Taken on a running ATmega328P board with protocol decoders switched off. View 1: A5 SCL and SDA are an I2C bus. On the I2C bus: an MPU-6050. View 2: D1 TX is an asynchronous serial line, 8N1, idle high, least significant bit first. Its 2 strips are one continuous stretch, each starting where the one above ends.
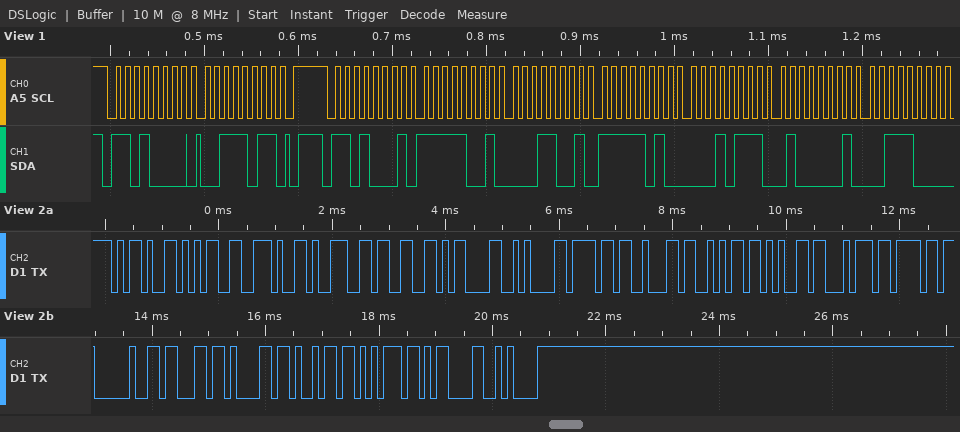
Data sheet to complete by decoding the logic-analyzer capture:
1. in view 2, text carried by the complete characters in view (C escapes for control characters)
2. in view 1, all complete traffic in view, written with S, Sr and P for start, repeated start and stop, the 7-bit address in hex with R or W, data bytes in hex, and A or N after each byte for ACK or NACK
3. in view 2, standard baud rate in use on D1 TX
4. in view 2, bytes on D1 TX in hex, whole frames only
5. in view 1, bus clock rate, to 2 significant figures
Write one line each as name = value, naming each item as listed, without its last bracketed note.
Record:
in view 2, text carried by the complete characters in view = "-5.93\r\nobjeto caiu\r\n"
in view 1, all complete traffic in view, written with S, Sr and P for start, repeated start and stop, the 7-bit address in hex with R or W, data bytes in hex, and A or N after each byte for ACK or NACK = S 68W A 3B A P S 68R A F9 A 19 A FA A 17 A 41 A 38 A
in view 2, standard baud rate in use on D1 TX = 9600 baud
in view 2, bytes on D1 TX in hex, whole frames only = 2D 35 2E 39 33 0D 0A 6F 62 6A 65 74 6F 20 63 61 69 75 0D 0A
in view 1, bus clock rate, to 2 significant figures = 100 kHz
